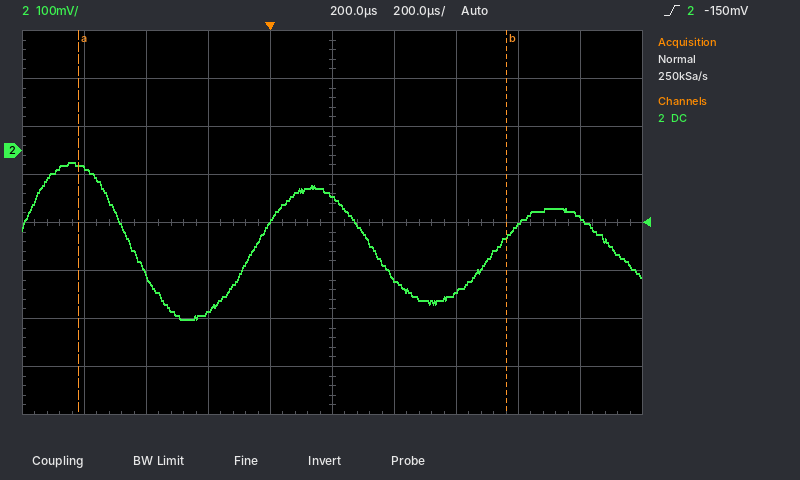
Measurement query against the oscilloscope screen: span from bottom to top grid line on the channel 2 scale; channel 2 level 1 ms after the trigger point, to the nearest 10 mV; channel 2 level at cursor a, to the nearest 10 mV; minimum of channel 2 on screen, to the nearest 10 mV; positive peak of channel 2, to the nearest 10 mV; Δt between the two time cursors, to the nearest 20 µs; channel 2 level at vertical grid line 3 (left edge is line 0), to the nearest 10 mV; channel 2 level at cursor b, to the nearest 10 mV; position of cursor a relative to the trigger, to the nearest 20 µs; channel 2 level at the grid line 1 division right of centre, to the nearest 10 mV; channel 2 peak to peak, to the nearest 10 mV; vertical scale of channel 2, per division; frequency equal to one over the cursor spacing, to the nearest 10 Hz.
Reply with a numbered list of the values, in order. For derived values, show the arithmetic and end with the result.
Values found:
1. 800 mV
2. -140 mV
3. -30 mV
4. -350 mV
5. -20 mV
6. 1.38 ms
7. -340 mV
8. -180 mV
9. -620 µs
10. -270 mV
11. -20 mV − (-350 mV) = 330 mV
12. 100 mV
13. 1 / 1.38 ms ≈ 720 Hz
